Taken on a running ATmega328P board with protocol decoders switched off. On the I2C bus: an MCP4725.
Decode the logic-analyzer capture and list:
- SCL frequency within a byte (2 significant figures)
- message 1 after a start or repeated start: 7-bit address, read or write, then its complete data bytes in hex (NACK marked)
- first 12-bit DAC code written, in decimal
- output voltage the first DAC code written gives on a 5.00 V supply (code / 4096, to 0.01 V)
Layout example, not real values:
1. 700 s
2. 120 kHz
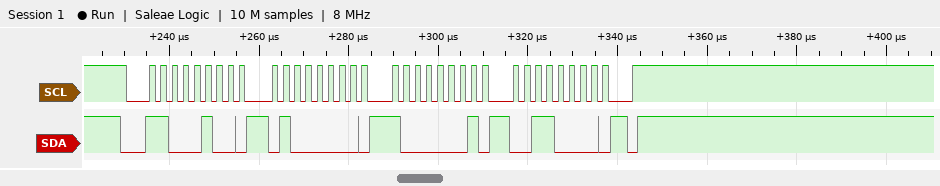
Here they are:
1. 400 kHz
2. 0x62 write: 40 81 30
3. 2067
4. 2.52 V
